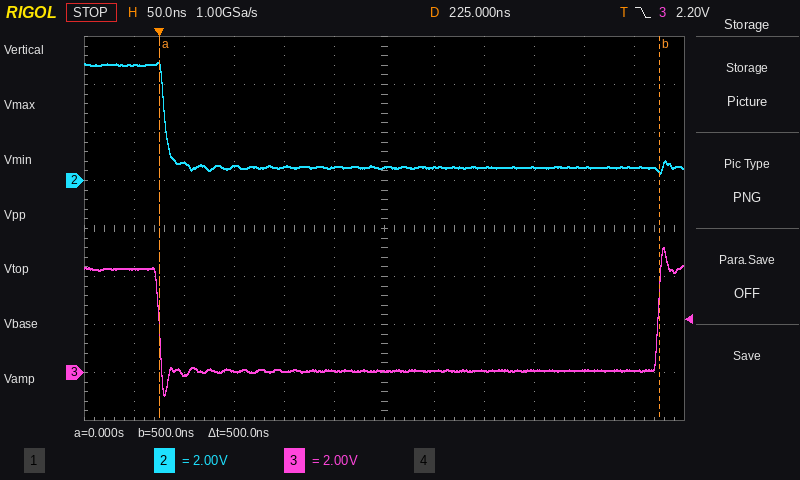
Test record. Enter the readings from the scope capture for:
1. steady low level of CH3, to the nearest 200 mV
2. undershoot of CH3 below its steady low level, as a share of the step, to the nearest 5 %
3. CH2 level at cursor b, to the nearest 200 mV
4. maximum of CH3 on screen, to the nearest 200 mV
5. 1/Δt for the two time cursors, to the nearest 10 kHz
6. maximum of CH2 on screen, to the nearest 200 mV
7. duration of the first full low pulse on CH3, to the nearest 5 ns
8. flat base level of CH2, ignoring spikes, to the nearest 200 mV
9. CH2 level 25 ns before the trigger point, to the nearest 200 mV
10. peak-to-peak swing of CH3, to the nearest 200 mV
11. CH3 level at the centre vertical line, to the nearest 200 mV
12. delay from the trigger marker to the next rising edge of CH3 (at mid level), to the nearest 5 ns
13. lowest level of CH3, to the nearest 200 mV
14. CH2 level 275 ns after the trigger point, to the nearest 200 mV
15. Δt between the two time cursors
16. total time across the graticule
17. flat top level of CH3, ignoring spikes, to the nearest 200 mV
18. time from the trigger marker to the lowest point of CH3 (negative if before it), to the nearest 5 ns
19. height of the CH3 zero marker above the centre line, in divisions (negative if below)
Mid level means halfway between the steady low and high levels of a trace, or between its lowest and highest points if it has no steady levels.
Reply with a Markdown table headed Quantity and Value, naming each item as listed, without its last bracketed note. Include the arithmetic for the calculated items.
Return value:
| Quantity | Value |
|---|---|
| steady low level of CH3, to the nearest 200 mV | 0.0 V |
| undershoot of CH3 below its steady low level, as a share of the step, to the nearest 5 % | 25 % |
| CH2 level at cursor b, to the nearest 200 mV | 400 mV |
| maximum of CH3 on screen, to the nearest 200 mV | 5.2 V |
| 1/Δt for the two time cursors, to the nearest 10 kHz | 1 / 500 ns ≈ 2.00 MHz |
| maximum of CH2 on screen, to the nearest 200 mV | 5.0 V |
| duration of the first full low pulse on CH3, to the nearest 5 ns | 500 ns |
| flat base level of CH2, ignoring spikes, to the nearest 200 mV | 600 mV |
| CH2 level 25 ns before the trigger point, to the nearest 200 mV | 4.8 V |
| peak-to-peak swing of CH3, to the nearest 200 mV | 5.2 V − (-1.0 V) = 6.2 V |
| CH3 level at the centre vertical line, to the nearest 200 mV | 0.0 V |
| delay from the trigger marker to the next rising edge of CH3 (at mid level), to the nearest 5 ns | 500 ns |
| lowest level of CH3, to the nearest 200 mV | -1.0 V |
| CH2 level 275 ns after the trigger point, to the nearest 200 mV | 600 mV |
| Δt between the two time cursors | 500 ns |
| total time across the graticule | 600 ns |
| flat top level of CH3, ignoring spikes, to the nearest 200 mV | 4.4 V |
| time from the trigger marker to the lowest point of CH3 (negative if before it), to the nearest 5 ns | +5 ns |
| height of the CH3 zero marker above the centre line, in divisions | -3.0 div |
